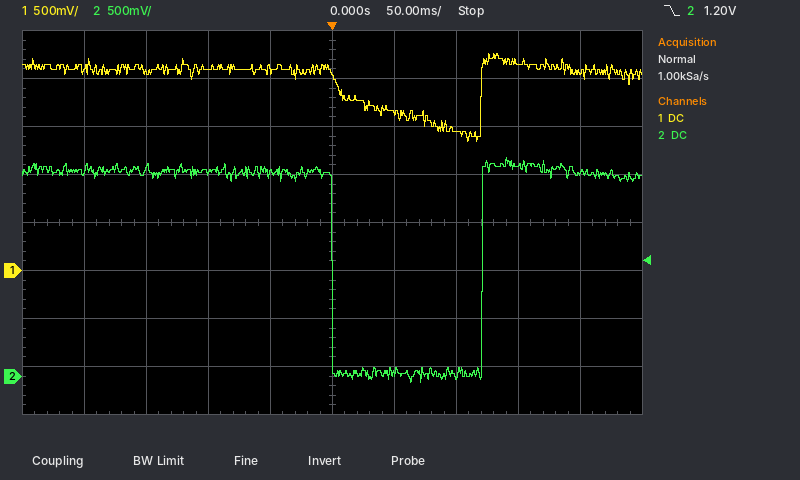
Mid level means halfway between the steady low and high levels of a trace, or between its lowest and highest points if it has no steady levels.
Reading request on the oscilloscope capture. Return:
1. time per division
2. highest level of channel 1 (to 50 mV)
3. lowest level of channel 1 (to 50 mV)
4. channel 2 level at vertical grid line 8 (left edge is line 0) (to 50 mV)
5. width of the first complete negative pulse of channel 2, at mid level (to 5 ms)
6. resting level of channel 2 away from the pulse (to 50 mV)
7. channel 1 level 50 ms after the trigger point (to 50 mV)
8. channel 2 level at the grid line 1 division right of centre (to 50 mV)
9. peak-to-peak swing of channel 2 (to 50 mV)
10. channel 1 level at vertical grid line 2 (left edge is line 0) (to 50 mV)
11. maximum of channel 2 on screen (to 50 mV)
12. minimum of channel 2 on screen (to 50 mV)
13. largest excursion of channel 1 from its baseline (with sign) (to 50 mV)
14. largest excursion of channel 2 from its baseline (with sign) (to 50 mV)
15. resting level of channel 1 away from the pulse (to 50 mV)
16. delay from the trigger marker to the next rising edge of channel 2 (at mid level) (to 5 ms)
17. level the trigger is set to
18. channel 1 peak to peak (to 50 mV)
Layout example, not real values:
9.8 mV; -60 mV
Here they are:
50 ms; 2.25 V; 1.35 V; 2.20 V; 120 ms; 2.15 V; 1.65 V; 50 mV; 2.35 V; 2.05 V; 2.30 V; -50 mV; -750 mV; -2.20 V; 2.10 V; 120 ms; 1.20 V; 900 mV
